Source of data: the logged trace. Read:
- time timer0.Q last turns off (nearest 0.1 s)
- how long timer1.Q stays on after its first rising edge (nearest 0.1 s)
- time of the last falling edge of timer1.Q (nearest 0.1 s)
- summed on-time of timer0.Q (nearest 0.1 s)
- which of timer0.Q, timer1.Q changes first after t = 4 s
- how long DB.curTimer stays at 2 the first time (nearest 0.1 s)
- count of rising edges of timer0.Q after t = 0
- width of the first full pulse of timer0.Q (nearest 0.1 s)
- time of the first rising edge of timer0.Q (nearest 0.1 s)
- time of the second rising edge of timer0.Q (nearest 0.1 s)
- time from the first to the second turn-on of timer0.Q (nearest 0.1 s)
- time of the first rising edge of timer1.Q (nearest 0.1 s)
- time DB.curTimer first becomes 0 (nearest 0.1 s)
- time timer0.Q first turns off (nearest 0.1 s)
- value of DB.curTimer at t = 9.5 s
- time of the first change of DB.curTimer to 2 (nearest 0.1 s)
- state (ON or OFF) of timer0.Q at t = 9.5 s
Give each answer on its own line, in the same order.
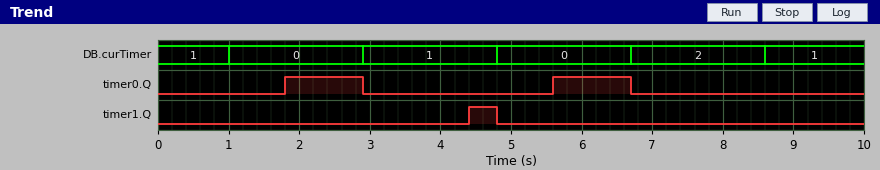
6.7 s
0.4 s
4.8 s
2.2 s
timer1.Q
1.9 s
2
1.1 s
1.8 s
5.6 s
3.8 s
4.4 s
1.0 s
2.9 s
1
6.7 s
OFF
